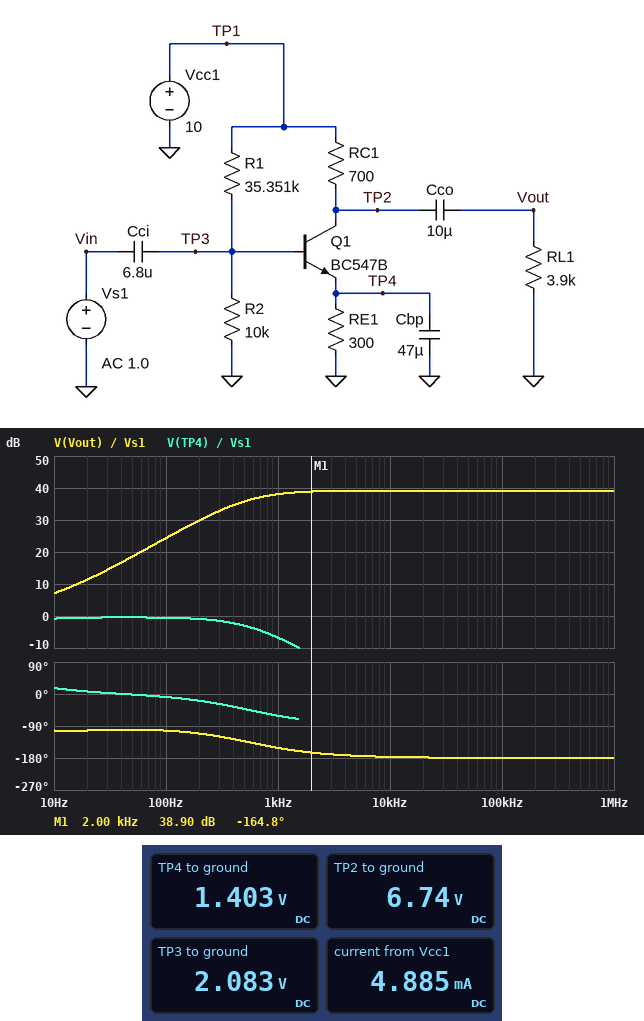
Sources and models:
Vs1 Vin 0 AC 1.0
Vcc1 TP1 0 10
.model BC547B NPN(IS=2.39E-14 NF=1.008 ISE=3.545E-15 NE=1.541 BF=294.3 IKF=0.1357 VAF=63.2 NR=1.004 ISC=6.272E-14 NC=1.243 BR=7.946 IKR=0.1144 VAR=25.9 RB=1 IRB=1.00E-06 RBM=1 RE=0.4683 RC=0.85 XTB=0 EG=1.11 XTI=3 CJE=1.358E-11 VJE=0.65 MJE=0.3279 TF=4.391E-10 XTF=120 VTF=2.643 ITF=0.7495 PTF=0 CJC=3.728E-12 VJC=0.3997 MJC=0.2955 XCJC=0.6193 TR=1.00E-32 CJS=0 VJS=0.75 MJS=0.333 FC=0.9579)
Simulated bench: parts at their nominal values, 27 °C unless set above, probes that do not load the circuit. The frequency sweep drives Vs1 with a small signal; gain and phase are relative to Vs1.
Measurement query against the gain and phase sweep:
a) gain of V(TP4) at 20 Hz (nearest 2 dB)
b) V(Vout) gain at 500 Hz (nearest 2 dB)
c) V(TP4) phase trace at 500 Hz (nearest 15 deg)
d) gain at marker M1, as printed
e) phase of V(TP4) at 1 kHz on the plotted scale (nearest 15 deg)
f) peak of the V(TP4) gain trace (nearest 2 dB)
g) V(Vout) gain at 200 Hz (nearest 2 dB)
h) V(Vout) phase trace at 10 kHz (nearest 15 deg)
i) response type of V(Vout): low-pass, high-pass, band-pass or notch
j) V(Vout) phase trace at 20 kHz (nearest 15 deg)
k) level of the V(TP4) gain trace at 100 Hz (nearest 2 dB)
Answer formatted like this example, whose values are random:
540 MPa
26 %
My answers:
0 dB
36 dB
-45 deg
38.90 dB
-60 deg
0 dB
30 dB
-180 deg
high-pass
-180 deg
0 dB
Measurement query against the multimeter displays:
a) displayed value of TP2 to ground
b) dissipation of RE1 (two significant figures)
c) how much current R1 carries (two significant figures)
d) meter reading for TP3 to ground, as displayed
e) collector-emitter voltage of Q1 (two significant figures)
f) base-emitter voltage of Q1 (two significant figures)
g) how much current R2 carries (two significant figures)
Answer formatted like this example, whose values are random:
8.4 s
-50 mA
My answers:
6.74 V
6.6 mW
220 µA
2.083 V
5.3 V
680 mV
210 µA
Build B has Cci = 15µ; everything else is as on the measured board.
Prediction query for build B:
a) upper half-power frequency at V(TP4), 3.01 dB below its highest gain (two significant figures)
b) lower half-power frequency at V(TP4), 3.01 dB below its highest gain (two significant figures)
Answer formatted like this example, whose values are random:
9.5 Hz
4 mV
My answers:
540 Hz
1.5 Hz
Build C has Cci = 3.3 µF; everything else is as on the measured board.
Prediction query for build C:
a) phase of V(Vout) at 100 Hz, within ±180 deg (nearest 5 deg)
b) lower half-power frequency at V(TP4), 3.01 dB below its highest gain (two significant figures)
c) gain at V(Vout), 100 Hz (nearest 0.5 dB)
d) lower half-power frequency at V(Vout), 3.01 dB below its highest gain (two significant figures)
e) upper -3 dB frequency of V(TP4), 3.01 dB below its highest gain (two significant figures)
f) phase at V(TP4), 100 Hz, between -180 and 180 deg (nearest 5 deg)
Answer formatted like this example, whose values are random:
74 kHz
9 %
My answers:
-100 deg
6.3 Hz
24.0 dB
560 Hz
570 Hz
-5 deg
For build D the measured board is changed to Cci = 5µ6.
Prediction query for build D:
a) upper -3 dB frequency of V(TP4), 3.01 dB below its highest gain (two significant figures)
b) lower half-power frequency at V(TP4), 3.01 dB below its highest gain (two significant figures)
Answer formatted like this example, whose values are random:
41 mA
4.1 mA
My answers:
560 Hz
3.8 Hz
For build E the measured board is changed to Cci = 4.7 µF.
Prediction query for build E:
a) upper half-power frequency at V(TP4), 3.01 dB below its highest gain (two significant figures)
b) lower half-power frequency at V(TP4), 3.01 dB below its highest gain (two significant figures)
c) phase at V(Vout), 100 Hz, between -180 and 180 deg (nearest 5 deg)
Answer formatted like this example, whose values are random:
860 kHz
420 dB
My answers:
560 Hz
4.5 Hz
-100 deg
